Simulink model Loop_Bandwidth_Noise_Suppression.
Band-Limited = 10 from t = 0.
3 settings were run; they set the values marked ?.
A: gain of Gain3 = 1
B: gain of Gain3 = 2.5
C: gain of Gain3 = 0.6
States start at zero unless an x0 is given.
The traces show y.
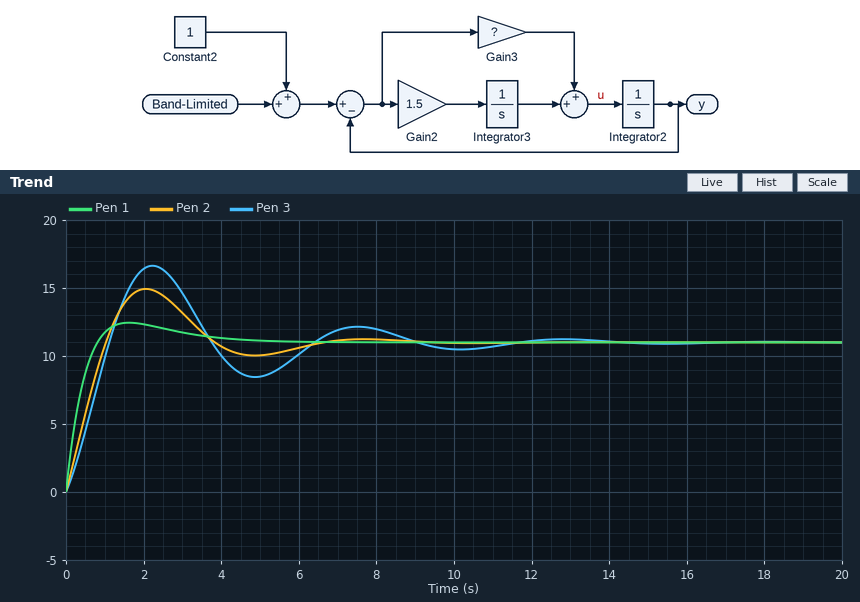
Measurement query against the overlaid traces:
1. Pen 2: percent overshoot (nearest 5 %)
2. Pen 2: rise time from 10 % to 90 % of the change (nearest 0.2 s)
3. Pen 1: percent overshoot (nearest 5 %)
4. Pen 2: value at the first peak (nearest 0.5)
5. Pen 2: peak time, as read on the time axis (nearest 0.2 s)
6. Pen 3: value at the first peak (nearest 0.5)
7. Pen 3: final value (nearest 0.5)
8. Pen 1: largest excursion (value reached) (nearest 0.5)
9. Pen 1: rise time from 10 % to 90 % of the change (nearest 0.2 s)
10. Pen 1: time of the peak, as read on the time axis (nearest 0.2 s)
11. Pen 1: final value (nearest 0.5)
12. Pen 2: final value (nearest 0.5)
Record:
35 %
0.8 s
15 %
15.0
2.0 s
16.5
11.0
12.5
0.6 s
1.6 s
11.0
11.0
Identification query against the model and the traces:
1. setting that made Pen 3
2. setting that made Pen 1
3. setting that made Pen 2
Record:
C
B
A
